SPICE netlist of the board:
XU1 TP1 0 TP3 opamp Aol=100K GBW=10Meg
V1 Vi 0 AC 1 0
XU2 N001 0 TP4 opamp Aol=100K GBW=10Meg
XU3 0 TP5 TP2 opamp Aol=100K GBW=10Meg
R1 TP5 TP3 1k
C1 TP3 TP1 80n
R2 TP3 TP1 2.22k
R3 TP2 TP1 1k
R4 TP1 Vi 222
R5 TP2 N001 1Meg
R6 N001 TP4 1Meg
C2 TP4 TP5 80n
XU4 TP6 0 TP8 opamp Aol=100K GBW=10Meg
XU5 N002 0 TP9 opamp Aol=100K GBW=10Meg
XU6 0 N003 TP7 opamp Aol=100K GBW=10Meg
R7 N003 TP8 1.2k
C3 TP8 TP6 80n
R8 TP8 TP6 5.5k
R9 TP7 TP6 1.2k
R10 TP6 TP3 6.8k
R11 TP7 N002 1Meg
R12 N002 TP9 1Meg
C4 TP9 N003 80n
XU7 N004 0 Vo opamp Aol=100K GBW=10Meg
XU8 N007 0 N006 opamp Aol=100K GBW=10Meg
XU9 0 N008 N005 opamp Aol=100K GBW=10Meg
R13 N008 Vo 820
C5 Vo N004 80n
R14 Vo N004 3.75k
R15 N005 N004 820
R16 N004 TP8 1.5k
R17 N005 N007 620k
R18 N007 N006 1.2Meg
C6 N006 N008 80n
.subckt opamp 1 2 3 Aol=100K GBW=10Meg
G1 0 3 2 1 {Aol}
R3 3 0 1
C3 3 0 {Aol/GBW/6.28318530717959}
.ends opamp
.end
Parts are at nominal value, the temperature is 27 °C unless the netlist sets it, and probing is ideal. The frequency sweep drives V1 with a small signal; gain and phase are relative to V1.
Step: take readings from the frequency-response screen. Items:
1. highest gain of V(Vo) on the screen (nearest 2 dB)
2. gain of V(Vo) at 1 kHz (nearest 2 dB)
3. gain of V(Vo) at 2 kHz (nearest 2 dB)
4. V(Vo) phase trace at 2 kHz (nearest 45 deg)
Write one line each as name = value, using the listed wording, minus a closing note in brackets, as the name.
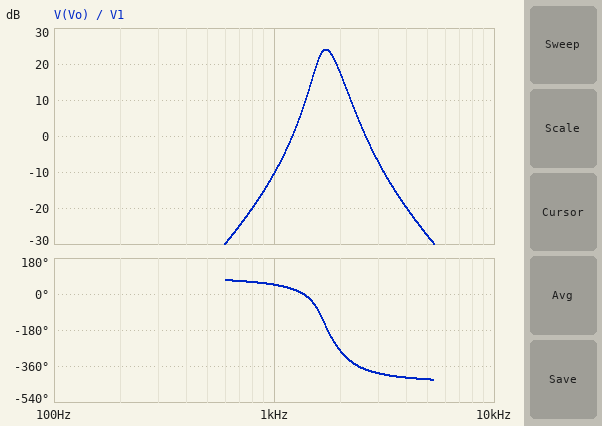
highest gain of V(Vo) on the screen = 24 dB
gain of V(Vo) at 1 kHz = -10 dB
gain of V(Vo) at 2 kHz = 18 dB
V(Vo) phase trace at 2 kHz = -270 deg
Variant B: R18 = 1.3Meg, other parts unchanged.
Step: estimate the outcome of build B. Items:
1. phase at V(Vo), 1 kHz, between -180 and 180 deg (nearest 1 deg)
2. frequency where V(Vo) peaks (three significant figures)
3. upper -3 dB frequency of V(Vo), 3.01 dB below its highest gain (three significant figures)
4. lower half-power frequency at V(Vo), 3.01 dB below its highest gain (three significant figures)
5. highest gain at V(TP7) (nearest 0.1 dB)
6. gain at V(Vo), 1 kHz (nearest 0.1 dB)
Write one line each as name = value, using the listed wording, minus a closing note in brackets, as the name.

phase at V(Vo), 1 kHz, between -180 and 180 deg = 45 deg
frequency where V(Vo) peaks = 1.69 kHz
upper -3 dB frequency of V(Vo), 3.01 dB below its highest gain = 1.85 kHz
lower half-power frequency at V(Vo), 3.01 dB below its highest gain = 1.57 kHz
highest gain at V(TP7) = 16.0 dB
gain at V(Vo), 1 kHz = -9.5 dB
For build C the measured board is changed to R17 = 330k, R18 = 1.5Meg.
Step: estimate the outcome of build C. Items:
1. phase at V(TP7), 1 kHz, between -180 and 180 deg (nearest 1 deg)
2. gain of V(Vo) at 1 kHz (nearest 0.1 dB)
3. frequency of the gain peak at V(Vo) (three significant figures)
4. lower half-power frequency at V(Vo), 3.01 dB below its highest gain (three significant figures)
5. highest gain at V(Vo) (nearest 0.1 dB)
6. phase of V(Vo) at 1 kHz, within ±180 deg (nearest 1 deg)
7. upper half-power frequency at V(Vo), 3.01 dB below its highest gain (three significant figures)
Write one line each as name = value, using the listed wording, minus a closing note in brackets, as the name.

phase at V(TP7), 1 kHz, between -180 and 180 deg = 61 deg
gain of V(Vo) at 1 kHz = 0.3 dB
frequency of the gain peak at V(Vo) = 1.66 kHz
lower half-power frequency at V(Vo), 3.01 dB below its highest gain = 1.49 kHz
highest gain at V(Vo) = 18.2 dB
phase of V(Vo) at 1 kHz, within ±180 deg = 0 deg
upper half-power frequency at V(Vo), 3.01 dB below its highest gain = 1.85 kHz
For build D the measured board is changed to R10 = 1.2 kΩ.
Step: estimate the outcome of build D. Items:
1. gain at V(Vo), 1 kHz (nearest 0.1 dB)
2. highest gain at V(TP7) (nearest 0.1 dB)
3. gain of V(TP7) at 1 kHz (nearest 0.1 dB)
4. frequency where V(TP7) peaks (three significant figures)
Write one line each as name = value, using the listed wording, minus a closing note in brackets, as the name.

gain at V(Vo), 1 kHz = 4.6 dB
highest gain at V(TP7) = 31.1 dB
gain of V(TP7) at 1 kHz = 13.0 dB
frequency where V(TP7) peaks = 1.68 kHz
